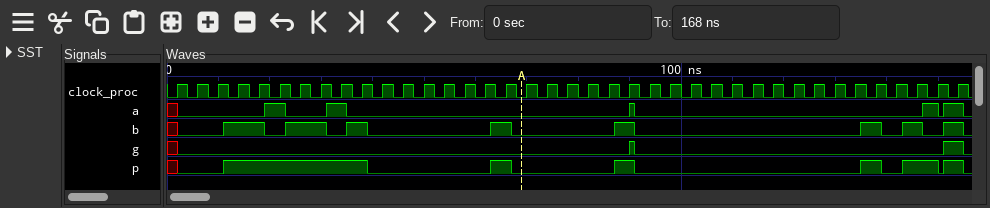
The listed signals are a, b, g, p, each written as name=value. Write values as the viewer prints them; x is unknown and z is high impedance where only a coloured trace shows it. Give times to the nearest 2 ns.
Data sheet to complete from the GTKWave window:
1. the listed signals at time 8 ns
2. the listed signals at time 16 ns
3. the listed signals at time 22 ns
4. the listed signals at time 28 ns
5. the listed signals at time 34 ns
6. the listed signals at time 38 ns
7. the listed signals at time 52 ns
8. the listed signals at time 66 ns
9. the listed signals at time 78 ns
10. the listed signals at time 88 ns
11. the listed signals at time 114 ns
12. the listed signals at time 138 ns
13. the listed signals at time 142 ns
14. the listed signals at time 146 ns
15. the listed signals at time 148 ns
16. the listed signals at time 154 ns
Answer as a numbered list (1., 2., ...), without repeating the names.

1. a=0, b=0, g=0, p=0
2. a=0, b=1, g=0, p=1
3. a=1, b=0, g=0, p=1
4. a=0, b=1, g=0, p=1
5. a=1, b=0, g=0, p=1
6. a=0, b=1, g=0, p=1
7. a=0, b=0, g=0, p=0
8. a=0, b=1, g=0, p=1
9. a=0, b=0, g=0, p=0
10. a=0, b=1, g=0, p=1
11. a=0, b=0, g=0, p=0
12. a=0, b=1, g=0, p=1
13. a=0, b=0, g=0, p=0
14. a=0, b=1, g=0, p=1
15. a=1, b=0, g=0, p=1
16. a=1, b=1, g=1, p=1
